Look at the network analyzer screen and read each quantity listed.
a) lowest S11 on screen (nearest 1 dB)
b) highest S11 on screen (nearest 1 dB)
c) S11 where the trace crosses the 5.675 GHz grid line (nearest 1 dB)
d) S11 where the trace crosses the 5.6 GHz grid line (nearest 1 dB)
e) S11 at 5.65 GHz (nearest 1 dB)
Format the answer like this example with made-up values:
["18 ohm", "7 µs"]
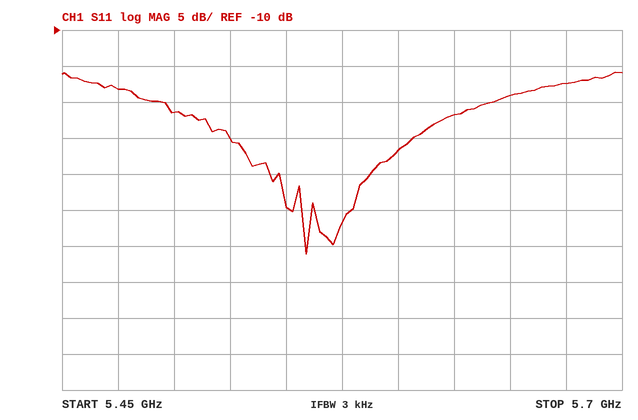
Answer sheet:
["-41 dB", "-16 dB", "-17 dB", "-27 dB", "-19 dB"]
